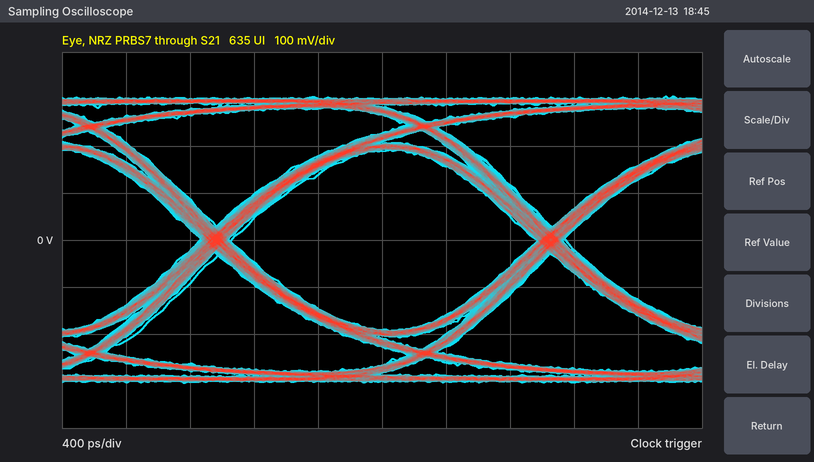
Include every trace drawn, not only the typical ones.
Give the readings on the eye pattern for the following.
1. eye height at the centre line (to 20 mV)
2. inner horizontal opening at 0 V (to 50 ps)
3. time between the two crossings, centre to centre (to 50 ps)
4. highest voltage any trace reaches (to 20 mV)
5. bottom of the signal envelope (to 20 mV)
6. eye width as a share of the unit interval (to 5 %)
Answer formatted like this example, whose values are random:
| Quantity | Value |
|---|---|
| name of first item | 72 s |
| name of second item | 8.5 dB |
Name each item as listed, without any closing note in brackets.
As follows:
| Quantity | Value |
|---|---|
| eye height at the centre line | 380 mV |
| inner horizontal opening at 0 V | 1.90 ns |
| time between the two crossings, centre to centre | 2.10 ns |
| highest voltage any trace reaches | 300 mV |
| bottom of the signal envelope | -300 mV |
| eye width as a share of the unit interval | 90 % |
